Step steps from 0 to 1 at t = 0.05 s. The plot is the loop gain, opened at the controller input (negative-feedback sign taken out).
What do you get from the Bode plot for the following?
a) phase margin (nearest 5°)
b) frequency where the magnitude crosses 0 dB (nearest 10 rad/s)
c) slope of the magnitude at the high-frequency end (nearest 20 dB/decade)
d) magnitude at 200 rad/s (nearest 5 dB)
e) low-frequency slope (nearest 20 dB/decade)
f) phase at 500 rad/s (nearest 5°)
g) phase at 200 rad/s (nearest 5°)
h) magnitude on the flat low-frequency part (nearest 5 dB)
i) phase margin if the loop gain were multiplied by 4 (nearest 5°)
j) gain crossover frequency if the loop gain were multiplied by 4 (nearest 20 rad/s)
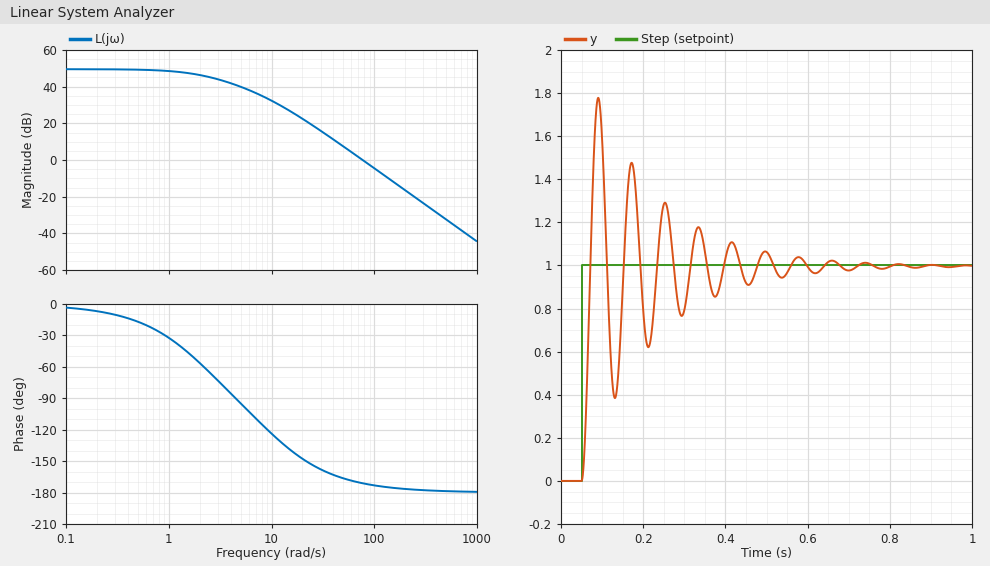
10°
80 rad/s
-40 dB/decade
-15 dB
0 dB/decade
-180°
-175°
50 dB
5°
160 rad/s
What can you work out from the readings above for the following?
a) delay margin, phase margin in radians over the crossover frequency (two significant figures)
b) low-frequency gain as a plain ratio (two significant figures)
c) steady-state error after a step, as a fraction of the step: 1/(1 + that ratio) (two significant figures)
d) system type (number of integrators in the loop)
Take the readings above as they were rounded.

0.0022 s
320
0.0031
0
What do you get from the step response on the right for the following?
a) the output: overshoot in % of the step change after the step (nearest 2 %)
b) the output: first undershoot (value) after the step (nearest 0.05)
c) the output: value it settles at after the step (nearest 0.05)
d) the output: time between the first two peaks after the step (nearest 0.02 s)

78 %
0.40
1.00
0.08 s
